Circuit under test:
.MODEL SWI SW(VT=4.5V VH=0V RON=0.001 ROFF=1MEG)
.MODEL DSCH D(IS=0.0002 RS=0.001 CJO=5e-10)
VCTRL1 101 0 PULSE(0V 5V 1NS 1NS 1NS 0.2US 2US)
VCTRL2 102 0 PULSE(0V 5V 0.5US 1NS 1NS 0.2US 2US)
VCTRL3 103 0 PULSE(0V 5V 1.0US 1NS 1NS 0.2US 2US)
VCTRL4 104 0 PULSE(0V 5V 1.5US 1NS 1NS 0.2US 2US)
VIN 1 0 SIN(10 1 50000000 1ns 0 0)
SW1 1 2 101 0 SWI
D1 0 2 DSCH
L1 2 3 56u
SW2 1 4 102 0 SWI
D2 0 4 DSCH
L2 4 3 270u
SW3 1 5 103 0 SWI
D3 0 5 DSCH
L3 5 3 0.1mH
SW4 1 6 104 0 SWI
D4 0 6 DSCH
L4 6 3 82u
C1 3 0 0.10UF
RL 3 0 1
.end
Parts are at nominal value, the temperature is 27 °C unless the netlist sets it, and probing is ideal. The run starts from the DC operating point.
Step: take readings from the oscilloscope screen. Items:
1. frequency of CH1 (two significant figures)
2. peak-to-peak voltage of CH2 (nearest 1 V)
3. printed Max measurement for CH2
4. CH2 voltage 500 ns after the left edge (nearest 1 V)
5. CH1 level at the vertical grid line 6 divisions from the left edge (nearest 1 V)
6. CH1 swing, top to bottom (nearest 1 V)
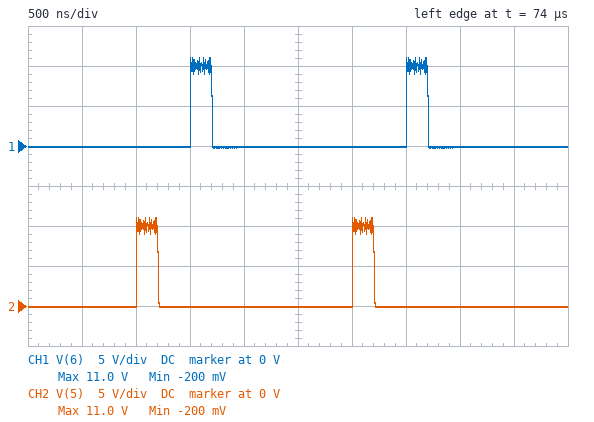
500 kHz
11 V
11.0 V
0 V
0 V
11 V
